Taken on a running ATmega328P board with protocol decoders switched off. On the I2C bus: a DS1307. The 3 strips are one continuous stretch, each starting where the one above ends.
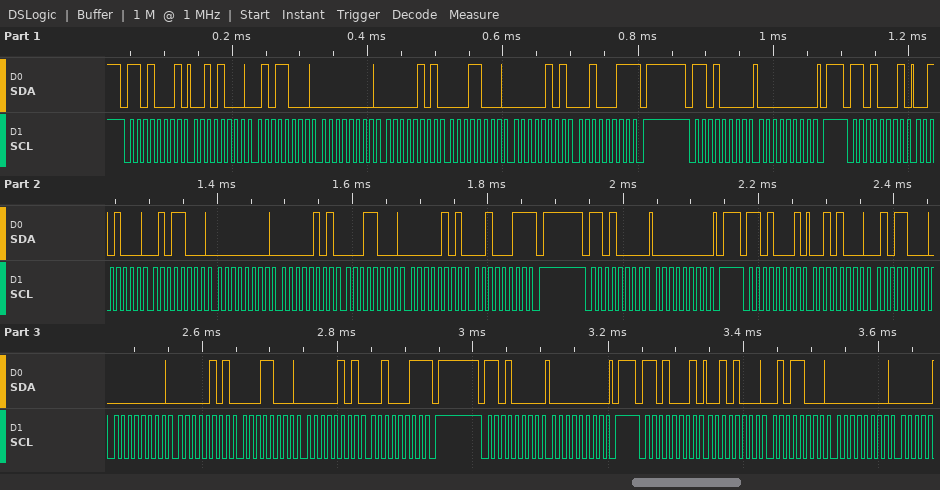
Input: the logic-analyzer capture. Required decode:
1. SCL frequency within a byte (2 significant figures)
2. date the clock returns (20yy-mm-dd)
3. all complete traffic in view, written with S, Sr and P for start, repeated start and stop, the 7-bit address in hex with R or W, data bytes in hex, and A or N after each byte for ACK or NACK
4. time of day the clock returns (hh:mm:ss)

100 kHz
2023-05-18
S 68R A 28 A 58 A 00 A 05 A 18 A 05 A 23 N P S 68W A 00 A P S 68R A 28 A 58 A 00 A 05 A 18 A 05 A 23 N P S 68W A 00 A P S 68R A 28 A 58 A 00 A 05 A 18 A 05 A 23 N P S 68W A 00 A P S 68R A 28 A 58 A 00 A
00:58:28
